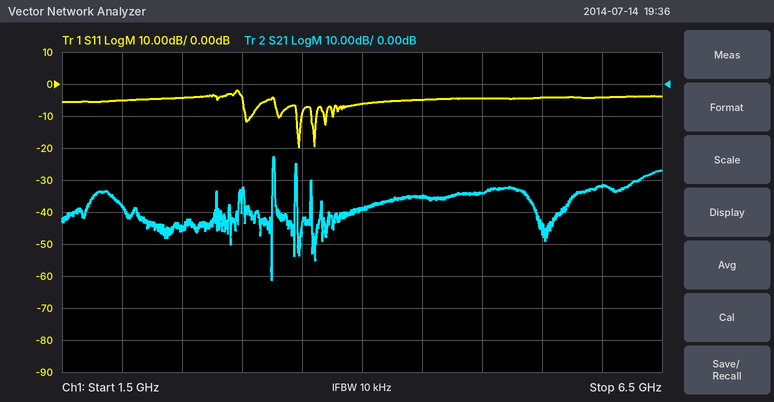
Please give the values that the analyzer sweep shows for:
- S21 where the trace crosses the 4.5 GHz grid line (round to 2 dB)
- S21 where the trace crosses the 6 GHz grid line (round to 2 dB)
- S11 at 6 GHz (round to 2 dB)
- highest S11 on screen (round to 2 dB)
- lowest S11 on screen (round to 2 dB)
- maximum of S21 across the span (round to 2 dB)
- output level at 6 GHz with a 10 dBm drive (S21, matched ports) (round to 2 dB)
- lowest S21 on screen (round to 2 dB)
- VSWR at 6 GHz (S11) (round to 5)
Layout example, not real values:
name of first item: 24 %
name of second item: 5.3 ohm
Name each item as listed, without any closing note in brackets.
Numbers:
S21 where the trace crosses the 4.5 GHz grid line: -36 dB
S21 where the trace crosses the 6 GHz grid line: -32 dB
S11 at 6 GHz: -4 dB
highest S11 on screen: -2 dB
lowest S11 on screen: -20 dB
maximum of S21 across the span: -22 dB
output level at 6 GHz with a 10 dBm drive (S21, matched ports): -22 dBm
lowest S21 on screen: -62 dB
VSWR at 6 GHz (S11): 5
